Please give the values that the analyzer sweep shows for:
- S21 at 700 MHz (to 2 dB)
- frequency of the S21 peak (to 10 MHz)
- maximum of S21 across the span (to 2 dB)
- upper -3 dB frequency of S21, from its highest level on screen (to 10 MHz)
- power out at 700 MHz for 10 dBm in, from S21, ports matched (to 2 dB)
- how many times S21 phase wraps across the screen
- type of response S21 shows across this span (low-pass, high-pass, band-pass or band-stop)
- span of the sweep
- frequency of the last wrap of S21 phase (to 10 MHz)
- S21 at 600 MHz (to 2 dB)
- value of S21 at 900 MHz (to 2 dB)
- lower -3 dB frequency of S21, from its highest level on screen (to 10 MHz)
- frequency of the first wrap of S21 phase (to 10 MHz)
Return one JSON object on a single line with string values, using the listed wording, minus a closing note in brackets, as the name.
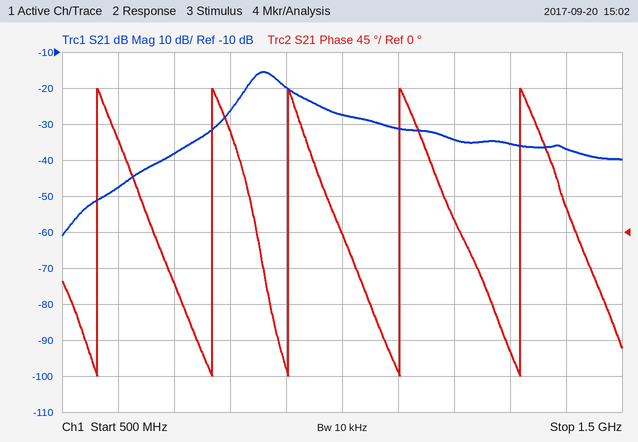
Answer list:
{"S21 at 700 MHz": "-38 dB", "frequency of the S21 peak": "860 MHz", "maximum of S21 across the span": "-16 dB", "upper -3 dB frequency of S21, from its highest level on screen": "890 MHz", "power out at 700 MHz for 10 dBm in, from S21, ports matched": "-28 dBm", "how many times S21 phase wraps across the screen": "5", "type of response S21 shows across this span": "band-pass", "span of the sweep": "1 GHz", "frequency of the last wrap of S21 phase": "1.32 GHz", "S21 at 600 MHz": "-48 dB", "value of S21 at 900 MHz": "-20 dB", "lower -3 dB frequency of S21, from its highest level on screen": "840 MHz", "frequency of the first wrap of S21 phase": "560 MHz"}
